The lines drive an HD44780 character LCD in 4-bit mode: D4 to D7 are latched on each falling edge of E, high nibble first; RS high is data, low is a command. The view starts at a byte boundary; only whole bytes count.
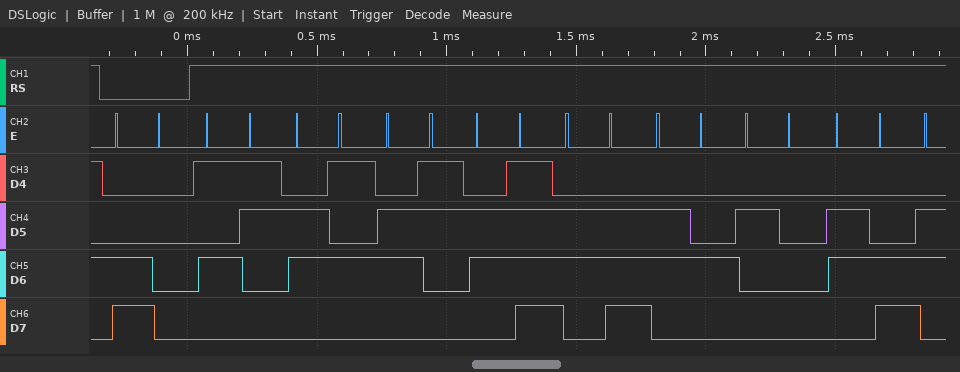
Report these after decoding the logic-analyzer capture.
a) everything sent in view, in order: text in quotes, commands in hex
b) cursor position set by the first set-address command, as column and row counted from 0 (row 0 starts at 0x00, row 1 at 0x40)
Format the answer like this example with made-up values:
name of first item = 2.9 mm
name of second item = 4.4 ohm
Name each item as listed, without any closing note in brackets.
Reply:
everything sent in view, in order: text in quotes, commands in hex = 0xC0 "Second l"
cursor position set by the first set-address command, as column and row counted from 0 = column 0, row 1
